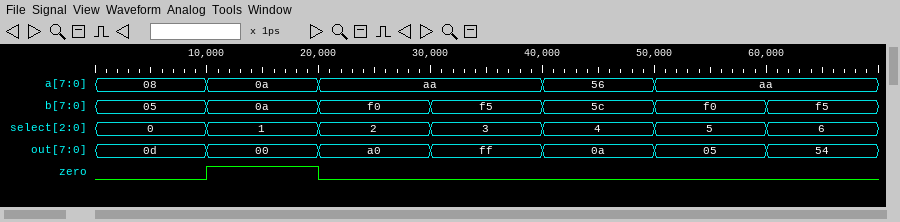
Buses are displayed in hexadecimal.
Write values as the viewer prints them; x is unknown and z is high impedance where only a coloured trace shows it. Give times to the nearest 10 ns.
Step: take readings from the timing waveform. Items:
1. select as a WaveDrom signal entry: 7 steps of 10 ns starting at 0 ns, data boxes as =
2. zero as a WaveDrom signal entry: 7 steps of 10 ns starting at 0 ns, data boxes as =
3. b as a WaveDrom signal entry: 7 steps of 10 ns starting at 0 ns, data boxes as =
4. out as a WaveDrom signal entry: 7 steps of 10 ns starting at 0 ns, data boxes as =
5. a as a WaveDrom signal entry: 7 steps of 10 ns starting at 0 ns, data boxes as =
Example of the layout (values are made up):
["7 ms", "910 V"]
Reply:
["{name: 'select', wave: '=======', data: '0 1 2 3 4 5 6'}", "{name: 'zero', wave: '010....'}", "{name: 'b', wave: '=======', data: '05 0a f0 f5 5c f0 f5'}", "{name: 'out', wave: '=======', data: '0d 00 a0 ff 0a 05 54'}", "{name: 'a', wave: '===.==.', data: '08 0a aa 56 aa'}"]
